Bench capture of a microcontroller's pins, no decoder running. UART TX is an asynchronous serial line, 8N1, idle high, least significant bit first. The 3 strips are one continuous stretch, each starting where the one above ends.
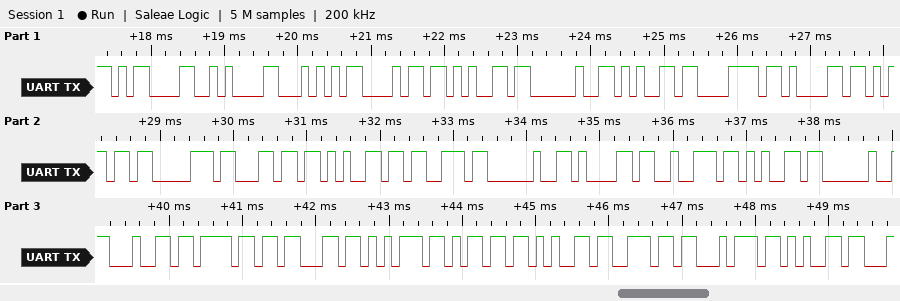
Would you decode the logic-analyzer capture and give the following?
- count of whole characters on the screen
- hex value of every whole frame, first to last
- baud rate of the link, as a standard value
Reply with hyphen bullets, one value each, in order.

- 28
- 0D 0A 54 68 65 20 65 78 61 6D 70 6C 65 73 20 61 72 65 20 64 6F 63 75 6D 65 6E 74 65
- 9600 baud
